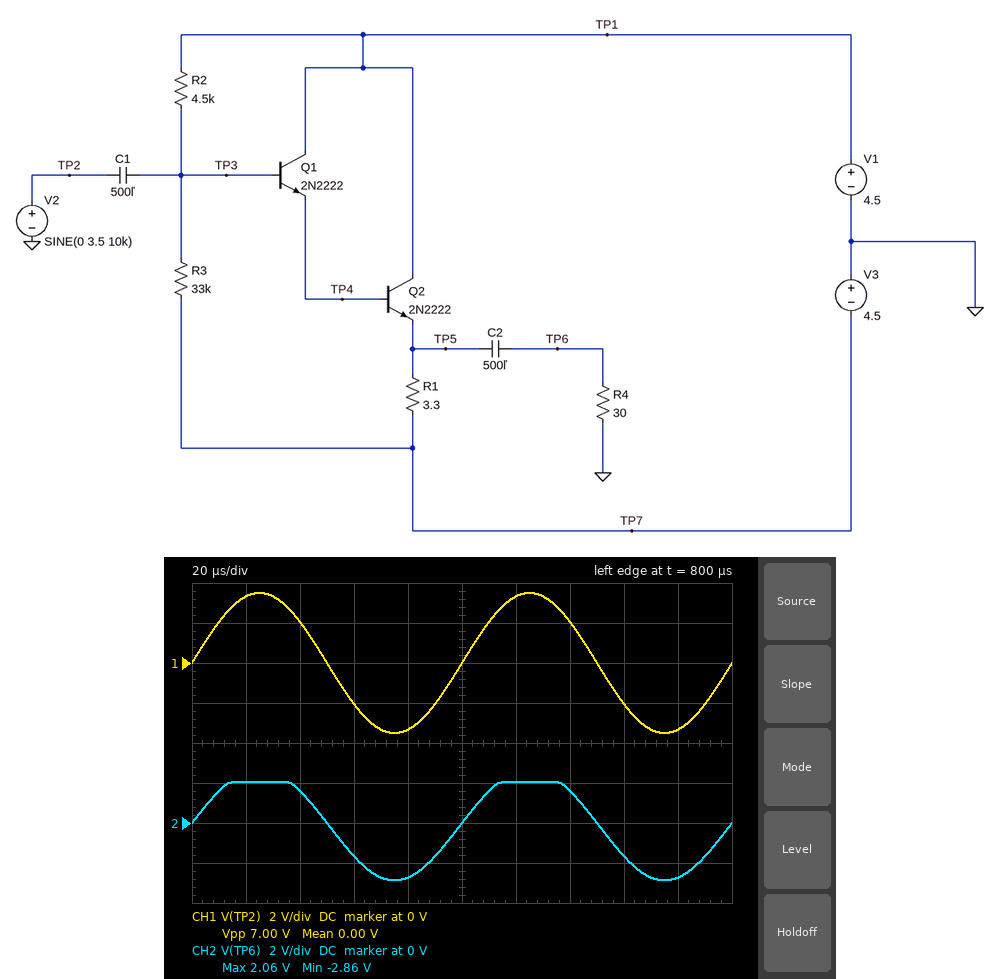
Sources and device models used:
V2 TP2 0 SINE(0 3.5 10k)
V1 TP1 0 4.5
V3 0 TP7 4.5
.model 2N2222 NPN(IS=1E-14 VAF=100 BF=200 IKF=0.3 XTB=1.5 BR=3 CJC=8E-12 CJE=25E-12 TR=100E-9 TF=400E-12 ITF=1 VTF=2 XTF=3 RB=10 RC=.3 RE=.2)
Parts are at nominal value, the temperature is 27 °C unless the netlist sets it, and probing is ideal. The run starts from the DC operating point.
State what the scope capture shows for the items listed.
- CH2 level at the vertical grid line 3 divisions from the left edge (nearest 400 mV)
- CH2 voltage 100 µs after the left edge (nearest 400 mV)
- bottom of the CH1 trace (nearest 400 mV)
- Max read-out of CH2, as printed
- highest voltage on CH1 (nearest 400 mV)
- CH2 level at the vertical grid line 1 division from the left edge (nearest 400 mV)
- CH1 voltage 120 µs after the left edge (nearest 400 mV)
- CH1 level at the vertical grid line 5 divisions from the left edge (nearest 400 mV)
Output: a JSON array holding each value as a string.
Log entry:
["-1.6 V", "0 V", "-3.6 V", "2.06 V", "3.6 V", "2.0 V", "3.2 V", "0 V"]
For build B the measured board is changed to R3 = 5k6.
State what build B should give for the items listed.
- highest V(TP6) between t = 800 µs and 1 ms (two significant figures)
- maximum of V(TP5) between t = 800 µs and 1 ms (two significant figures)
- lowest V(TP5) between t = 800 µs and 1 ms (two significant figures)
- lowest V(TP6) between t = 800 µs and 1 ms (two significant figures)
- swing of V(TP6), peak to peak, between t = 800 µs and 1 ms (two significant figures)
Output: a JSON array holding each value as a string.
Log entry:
["2.8 V", "1.2 V", "-4.2 V", "-2.6 V", "5.4 V"]
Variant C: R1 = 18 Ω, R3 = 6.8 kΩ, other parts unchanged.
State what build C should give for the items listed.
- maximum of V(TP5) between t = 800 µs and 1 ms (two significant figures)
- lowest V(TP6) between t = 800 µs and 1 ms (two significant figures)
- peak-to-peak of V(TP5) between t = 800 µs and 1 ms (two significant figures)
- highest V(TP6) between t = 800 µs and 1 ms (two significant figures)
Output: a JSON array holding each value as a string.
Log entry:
["2.7 V", "-2.4 V", "5.7 V", "3.3 V"]
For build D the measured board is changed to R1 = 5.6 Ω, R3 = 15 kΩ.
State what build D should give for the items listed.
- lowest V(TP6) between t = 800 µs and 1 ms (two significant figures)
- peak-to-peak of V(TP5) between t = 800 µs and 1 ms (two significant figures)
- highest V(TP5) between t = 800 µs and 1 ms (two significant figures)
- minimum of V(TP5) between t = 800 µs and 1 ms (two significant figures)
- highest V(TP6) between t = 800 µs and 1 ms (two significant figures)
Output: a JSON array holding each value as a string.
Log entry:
["-3.1 V", "5.8 V", "2.9 V", "-2.9 V", "2.7 V"]
